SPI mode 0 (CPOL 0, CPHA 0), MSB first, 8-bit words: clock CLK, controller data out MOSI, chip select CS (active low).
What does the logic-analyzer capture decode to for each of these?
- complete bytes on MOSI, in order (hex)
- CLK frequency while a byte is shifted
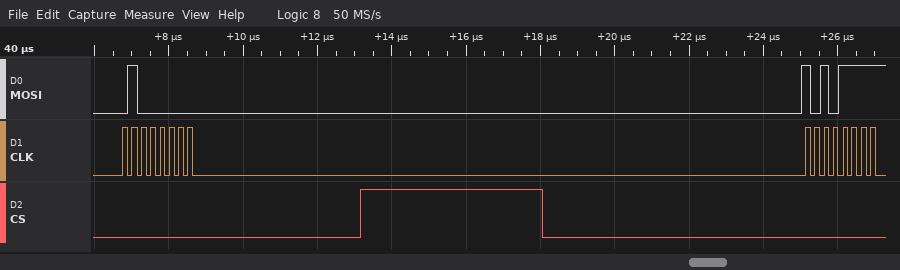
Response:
40 AF
4 MHz
